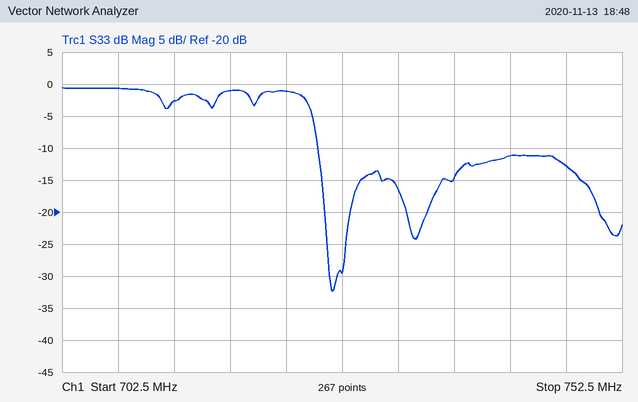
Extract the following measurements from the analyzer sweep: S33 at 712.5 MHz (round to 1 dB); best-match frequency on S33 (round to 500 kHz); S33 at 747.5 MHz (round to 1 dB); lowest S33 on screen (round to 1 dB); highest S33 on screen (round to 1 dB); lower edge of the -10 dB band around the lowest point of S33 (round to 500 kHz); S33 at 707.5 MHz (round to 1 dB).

-3 dB
726.5 MHz
-13 dB
-32 dB
-1 dB
725.5 MHz
-1 dB
